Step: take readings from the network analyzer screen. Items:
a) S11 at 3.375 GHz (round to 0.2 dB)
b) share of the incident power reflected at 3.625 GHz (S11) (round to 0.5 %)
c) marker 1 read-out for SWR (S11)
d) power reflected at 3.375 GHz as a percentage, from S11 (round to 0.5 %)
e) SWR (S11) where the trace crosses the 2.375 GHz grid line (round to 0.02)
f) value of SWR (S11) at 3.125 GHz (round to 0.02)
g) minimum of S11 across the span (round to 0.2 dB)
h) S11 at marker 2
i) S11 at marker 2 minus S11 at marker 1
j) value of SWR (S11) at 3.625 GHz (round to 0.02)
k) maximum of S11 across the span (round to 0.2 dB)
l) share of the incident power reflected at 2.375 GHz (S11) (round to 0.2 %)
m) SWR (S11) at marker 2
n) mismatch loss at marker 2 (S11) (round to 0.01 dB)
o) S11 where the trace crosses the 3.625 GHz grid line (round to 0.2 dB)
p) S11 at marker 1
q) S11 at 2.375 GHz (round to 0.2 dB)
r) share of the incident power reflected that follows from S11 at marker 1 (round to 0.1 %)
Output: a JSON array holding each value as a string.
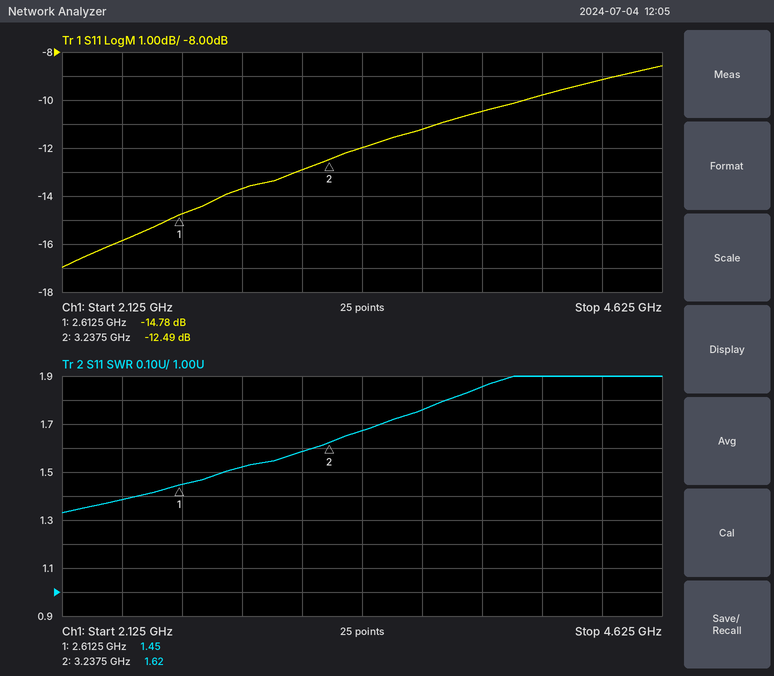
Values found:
["-12.0 dB", "7.5 %", "1.45", "6.5 %", "1.38", "1.58", "-17.0 dB", "-12.49 dB", "2.29 dB", "1.76", "-8.6 dB", "2.6 %", "1.62", "0.25 dB", "-11.2 dB", "-14.78 dB", "-15.8 dB", "3.3 %"]
